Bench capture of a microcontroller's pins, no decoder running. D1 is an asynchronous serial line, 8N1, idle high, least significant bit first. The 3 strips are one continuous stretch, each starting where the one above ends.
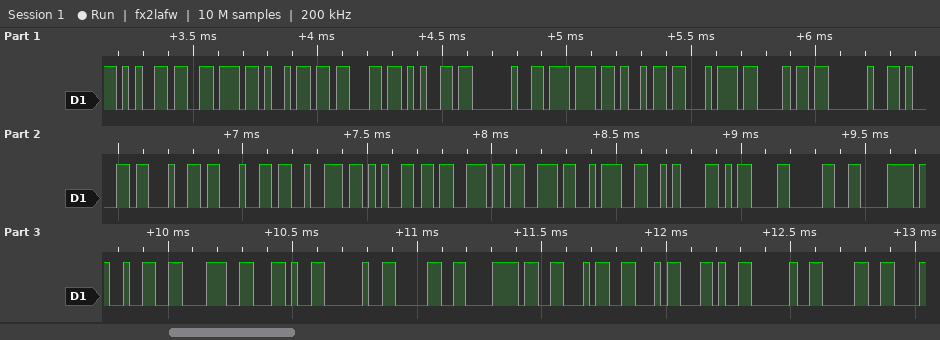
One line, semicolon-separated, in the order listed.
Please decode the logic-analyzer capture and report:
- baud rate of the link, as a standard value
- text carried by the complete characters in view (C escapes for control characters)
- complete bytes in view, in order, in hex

38400 baud; "evice with address:\n\r0x28, 0xFF, 0"; 65 76 69 63 65 20 77 69 74 68 20 61 64 64 72 65 73 73 3A 0A 0D 30 78 32 38 2C 20 30 78 46 46 2C 20 30
